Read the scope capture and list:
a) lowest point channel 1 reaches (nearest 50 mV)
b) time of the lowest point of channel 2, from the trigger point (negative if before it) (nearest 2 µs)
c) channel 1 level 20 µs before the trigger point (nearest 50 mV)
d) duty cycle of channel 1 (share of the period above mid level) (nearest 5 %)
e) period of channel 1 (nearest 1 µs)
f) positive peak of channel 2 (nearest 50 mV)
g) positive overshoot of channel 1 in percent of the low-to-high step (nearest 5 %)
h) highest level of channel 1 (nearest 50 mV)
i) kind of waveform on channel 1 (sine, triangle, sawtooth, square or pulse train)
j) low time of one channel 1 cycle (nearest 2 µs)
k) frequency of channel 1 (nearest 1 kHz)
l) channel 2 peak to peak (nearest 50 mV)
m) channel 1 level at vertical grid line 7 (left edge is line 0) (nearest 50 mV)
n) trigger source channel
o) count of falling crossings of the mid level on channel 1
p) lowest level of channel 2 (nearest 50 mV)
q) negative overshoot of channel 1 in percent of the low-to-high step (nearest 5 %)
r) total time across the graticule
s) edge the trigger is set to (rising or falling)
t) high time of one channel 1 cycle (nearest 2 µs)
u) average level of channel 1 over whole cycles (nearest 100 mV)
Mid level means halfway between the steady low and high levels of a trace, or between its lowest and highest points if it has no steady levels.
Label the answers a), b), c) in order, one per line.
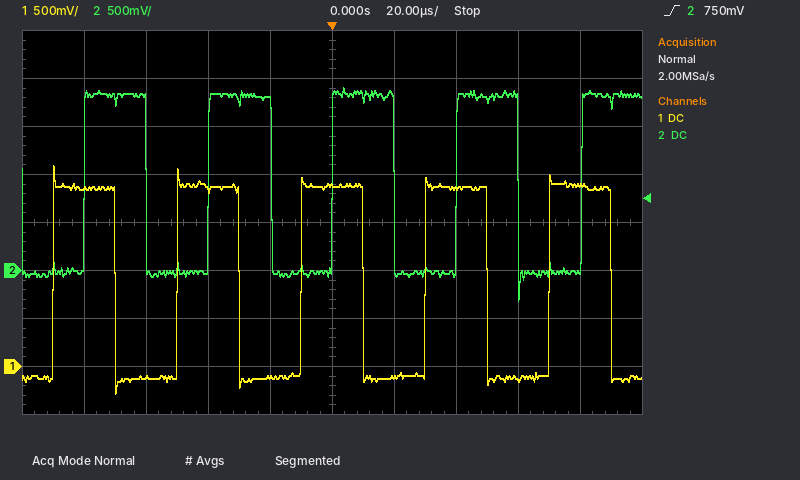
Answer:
a) -300 mV
b) +60 µs
c) -100 mV
d) 50 %
e) 40 µs
f) 1.90 V
g) 10 %
h) 2.10 V
i) square
j) 20 µs
k) 25 kHz
l) 2.20 V
m) 1.85 V
n) channel 2
o) 5
p) -300 mV
q) 10 %
r) 200 µs
s) rising
t) 20 µs
u) 900 mV
